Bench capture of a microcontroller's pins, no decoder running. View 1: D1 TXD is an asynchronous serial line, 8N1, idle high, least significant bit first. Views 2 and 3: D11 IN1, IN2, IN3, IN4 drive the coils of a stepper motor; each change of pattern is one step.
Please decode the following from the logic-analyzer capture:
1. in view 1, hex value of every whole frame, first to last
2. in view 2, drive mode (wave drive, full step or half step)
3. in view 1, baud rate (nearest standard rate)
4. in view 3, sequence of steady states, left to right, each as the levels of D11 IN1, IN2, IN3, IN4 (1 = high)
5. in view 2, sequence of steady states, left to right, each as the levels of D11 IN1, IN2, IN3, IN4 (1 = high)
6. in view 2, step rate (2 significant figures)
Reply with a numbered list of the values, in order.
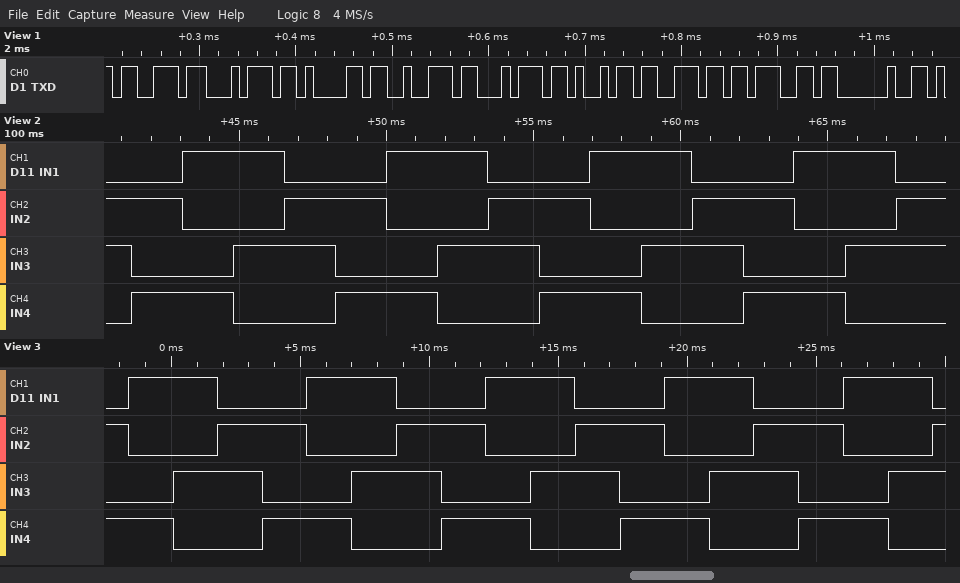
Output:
1. 73 74 61 72 74 69 6E 67 20
2. full step
3. 115200 baud
4. 0101 1001 1010 0110 0101 1001 1010 0110 0101 1001 1010 0110 0101 1001 1010 0110 0101 1001 1010 0110
5. 0110 0101 1001 1010 0110 0101 1001 1010 0110 0101 1001 1010 0110 0101 1001 1010 0110
6. 580 steps/s
